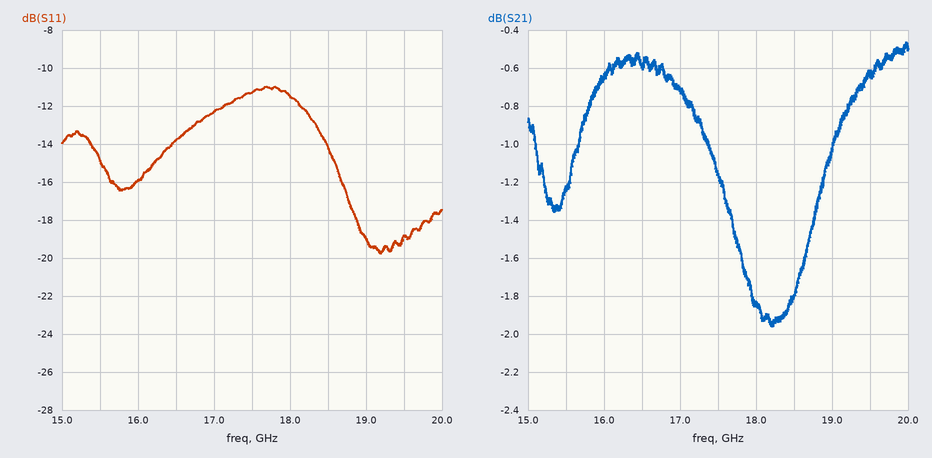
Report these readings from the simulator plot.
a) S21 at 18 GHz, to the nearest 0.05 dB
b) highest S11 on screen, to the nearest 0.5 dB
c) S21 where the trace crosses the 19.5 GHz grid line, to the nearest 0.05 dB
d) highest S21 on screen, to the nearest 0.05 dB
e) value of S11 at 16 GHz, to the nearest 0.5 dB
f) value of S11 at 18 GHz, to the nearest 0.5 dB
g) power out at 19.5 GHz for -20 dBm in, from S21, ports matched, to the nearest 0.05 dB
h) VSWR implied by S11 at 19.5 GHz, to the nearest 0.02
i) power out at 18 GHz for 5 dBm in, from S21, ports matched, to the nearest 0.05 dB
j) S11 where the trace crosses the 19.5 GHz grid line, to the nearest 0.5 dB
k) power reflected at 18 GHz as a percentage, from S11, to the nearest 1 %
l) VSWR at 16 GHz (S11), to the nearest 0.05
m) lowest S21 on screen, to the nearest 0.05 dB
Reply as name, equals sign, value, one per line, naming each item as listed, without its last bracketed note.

S21 at 18 GHz, to the nearest 0.05 dB = -1.85 dB
highest S11 on screen, to the nearest 0.5 dB = -11.0 dB
S21 where the trace crosses the 19.5 GHz grid line, to the nearest 0.05 dB = -0.65 dB
highest S21 on screen, to the nearest 0.05 dB = -0.45 dB
value of S11 at 16 GHz, to the nearest 0.5 dB = -16.0 dB
value of S11 at 18 GHz, to the nearest 0.5 dB = -11.5 dB
power out at 19.5 GHz for -20 dBm in, from S21, ports matched, to the nearest 0.05 dB = -20.65 dBm
VSWR implied by S11 at 19.5 GHz, to the nearest 0.02 = 1.26
power out at 18 GHz for 5 dBm in, from S21, ports matched, to the nearest 0.05 dB = 3.15 dBm
S11 where the trace crosses the 19.5 GHz grid line, to the nearest 0.5 dB = -19.0 dB
power reflected at 18 GHz as a percentage, from S11, to the nearest 1 % = 7 %
VSWR at 16 GHz (S11), to the nearest 0.05 = 1.40
lowest S21 on screen, to the nearest 0.05 dB = -1.95 dB
